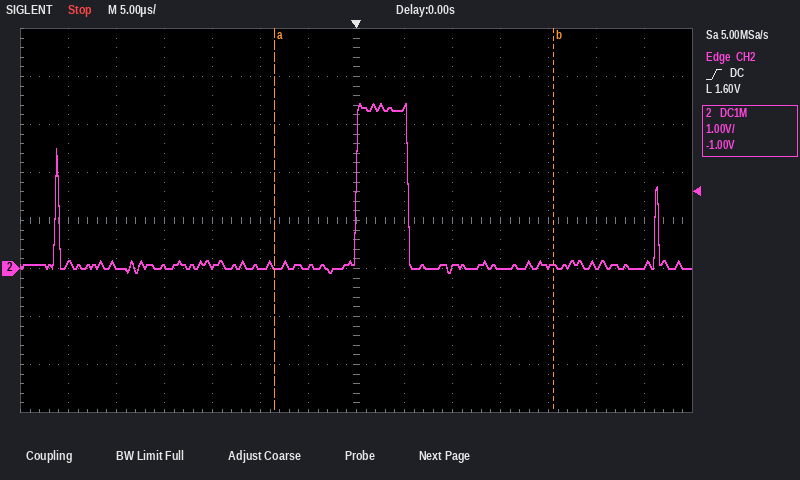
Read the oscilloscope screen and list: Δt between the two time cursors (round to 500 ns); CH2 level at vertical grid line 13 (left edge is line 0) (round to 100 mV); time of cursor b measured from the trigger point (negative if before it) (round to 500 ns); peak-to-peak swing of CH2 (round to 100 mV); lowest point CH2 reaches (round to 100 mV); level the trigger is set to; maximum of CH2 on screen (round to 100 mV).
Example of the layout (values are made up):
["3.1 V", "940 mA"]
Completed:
["29.0 µs", "0.0 V", "+20.5 µs", "3.5 V", "-100 mV", "1.60 V", "3.4 V"]
